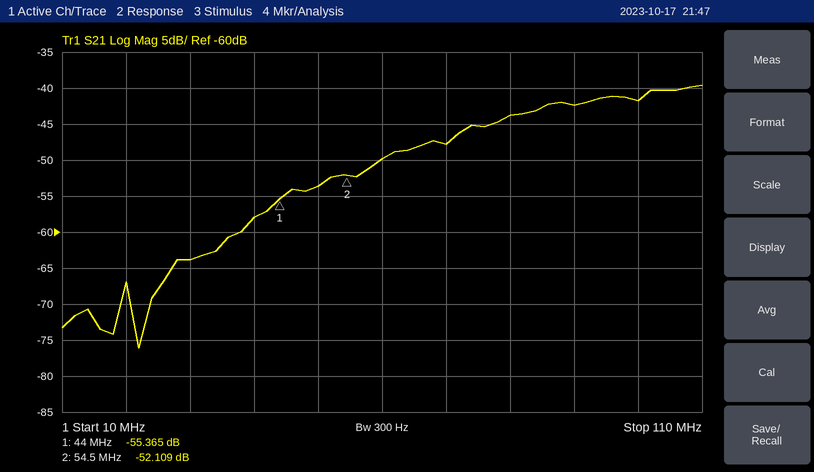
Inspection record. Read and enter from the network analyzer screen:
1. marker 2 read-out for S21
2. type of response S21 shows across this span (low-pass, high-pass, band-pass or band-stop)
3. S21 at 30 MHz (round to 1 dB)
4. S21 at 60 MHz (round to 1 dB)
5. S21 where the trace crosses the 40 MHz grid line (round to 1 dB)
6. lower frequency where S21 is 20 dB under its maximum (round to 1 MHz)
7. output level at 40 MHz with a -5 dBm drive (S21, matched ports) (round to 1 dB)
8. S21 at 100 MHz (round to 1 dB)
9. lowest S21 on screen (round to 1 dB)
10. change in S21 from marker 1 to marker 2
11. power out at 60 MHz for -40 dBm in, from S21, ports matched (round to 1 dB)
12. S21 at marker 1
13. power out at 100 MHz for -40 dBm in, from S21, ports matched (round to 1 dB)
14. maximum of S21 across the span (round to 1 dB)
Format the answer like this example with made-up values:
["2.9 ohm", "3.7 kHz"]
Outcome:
["-52.109 dB", "high-pass", "-64 dB", "-50 dB", "-58 dB", "38 MHz", "-63 dBm", "-42 dB", "-76 dB", "3.256 dB", "-90 dBm", "-55.365 dB", "-82 dBm", "-40 dB"]
